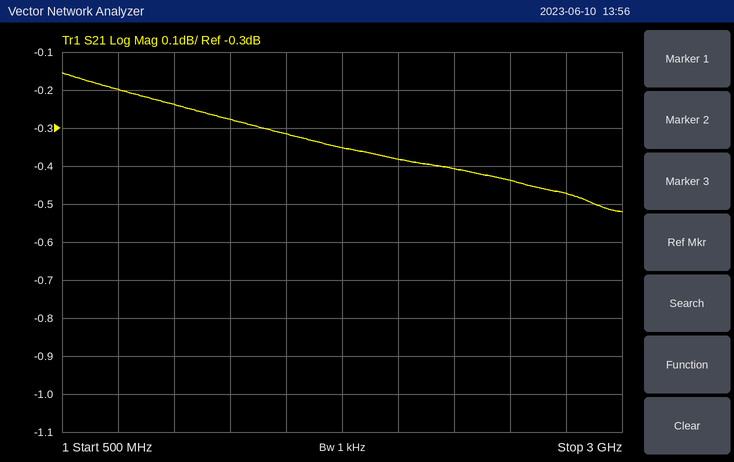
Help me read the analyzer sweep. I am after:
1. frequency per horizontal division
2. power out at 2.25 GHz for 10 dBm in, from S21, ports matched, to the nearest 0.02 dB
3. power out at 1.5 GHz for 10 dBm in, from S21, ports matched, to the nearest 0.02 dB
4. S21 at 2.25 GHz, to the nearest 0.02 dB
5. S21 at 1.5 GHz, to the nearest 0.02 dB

250 MHz
9.60 dBm
9.68 dBm
-0.40 dB
-0.32 dB
